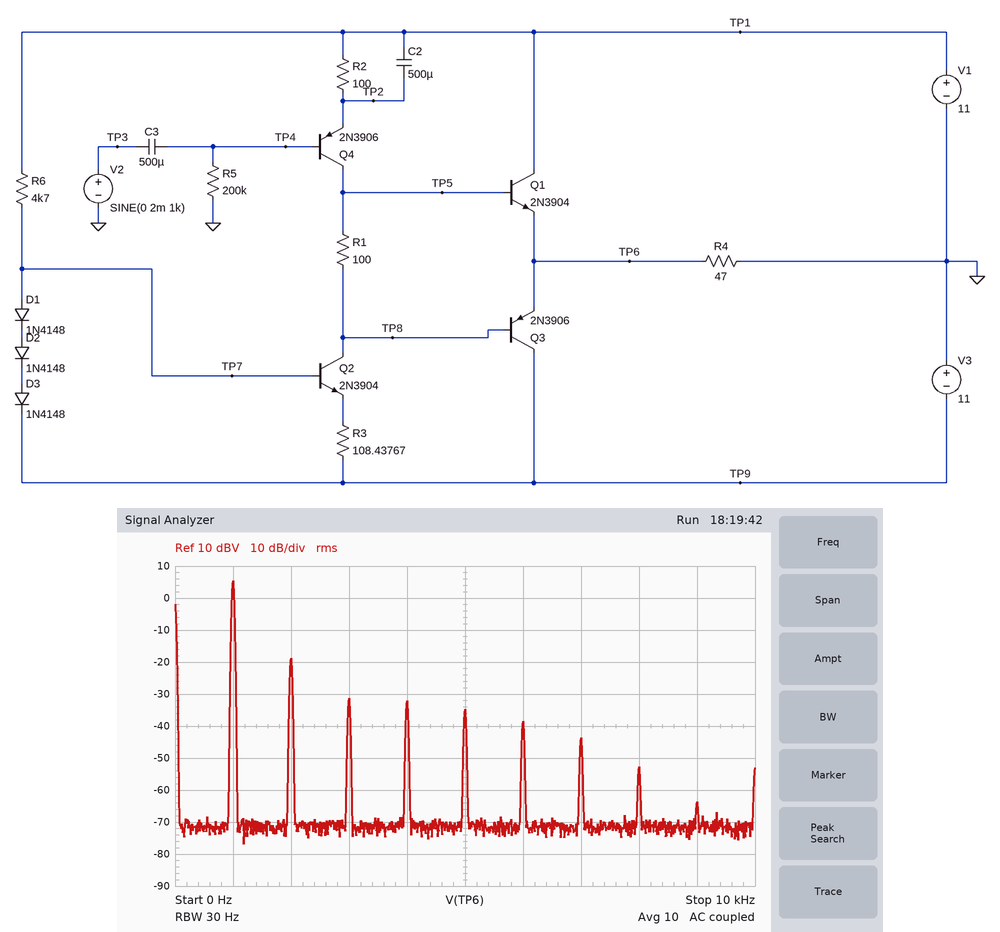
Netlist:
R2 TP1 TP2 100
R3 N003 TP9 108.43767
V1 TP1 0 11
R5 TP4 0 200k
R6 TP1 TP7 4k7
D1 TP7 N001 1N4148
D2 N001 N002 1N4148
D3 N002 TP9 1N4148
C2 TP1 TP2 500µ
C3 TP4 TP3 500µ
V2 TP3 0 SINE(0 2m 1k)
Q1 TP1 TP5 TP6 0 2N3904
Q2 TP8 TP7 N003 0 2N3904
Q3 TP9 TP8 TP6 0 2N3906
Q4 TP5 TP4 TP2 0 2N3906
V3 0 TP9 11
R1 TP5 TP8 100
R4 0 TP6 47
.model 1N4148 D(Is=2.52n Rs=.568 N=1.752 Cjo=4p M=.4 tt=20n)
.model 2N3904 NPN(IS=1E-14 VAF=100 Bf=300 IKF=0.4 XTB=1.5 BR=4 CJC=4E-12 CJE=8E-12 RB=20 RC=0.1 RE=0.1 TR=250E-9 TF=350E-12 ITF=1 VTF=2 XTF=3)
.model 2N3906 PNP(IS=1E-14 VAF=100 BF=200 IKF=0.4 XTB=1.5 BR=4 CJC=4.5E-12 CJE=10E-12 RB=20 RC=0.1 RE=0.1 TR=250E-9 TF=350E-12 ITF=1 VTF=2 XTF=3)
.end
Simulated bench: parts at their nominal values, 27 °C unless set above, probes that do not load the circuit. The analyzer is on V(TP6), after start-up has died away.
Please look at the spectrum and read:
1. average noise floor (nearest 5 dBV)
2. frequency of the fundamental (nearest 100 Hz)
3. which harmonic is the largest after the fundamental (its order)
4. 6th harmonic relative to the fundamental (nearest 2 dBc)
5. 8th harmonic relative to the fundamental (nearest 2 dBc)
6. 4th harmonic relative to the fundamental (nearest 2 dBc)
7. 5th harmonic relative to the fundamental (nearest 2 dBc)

-70 dBV
1.0 kHz
2
-44 dBc
-58 dBc
-38 dBc
-40 dBc
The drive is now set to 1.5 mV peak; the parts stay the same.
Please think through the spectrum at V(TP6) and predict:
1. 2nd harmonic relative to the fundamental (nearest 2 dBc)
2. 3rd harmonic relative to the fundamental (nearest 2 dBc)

-30 dBc
-60 dBc
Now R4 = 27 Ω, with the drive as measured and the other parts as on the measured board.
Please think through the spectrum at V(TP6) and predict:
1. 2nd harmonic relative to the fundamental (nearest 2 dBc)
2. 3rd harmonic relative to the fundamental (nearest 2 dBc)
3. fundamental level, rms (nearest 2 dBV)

-26 dBc
-50 dBc
2 dBV
